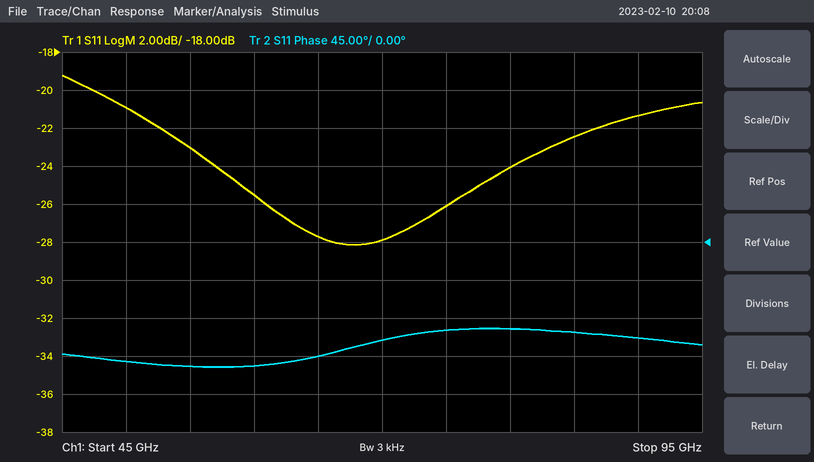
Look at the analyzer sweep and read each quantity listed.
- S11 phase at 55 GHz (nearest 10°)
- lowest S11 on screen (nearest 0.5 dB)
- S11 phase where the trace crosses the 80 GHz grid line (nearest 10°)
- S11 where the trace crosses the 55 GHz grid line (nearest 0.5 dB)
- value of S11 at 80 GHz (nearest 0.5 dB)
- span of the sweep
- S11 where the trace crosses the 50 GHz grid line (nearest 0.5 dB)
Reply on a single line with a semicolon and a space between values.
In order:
-150°; -28.0 dB; -100°; -23.0 dB; -24.0 dB; 50 GHz; -21.0 dB
